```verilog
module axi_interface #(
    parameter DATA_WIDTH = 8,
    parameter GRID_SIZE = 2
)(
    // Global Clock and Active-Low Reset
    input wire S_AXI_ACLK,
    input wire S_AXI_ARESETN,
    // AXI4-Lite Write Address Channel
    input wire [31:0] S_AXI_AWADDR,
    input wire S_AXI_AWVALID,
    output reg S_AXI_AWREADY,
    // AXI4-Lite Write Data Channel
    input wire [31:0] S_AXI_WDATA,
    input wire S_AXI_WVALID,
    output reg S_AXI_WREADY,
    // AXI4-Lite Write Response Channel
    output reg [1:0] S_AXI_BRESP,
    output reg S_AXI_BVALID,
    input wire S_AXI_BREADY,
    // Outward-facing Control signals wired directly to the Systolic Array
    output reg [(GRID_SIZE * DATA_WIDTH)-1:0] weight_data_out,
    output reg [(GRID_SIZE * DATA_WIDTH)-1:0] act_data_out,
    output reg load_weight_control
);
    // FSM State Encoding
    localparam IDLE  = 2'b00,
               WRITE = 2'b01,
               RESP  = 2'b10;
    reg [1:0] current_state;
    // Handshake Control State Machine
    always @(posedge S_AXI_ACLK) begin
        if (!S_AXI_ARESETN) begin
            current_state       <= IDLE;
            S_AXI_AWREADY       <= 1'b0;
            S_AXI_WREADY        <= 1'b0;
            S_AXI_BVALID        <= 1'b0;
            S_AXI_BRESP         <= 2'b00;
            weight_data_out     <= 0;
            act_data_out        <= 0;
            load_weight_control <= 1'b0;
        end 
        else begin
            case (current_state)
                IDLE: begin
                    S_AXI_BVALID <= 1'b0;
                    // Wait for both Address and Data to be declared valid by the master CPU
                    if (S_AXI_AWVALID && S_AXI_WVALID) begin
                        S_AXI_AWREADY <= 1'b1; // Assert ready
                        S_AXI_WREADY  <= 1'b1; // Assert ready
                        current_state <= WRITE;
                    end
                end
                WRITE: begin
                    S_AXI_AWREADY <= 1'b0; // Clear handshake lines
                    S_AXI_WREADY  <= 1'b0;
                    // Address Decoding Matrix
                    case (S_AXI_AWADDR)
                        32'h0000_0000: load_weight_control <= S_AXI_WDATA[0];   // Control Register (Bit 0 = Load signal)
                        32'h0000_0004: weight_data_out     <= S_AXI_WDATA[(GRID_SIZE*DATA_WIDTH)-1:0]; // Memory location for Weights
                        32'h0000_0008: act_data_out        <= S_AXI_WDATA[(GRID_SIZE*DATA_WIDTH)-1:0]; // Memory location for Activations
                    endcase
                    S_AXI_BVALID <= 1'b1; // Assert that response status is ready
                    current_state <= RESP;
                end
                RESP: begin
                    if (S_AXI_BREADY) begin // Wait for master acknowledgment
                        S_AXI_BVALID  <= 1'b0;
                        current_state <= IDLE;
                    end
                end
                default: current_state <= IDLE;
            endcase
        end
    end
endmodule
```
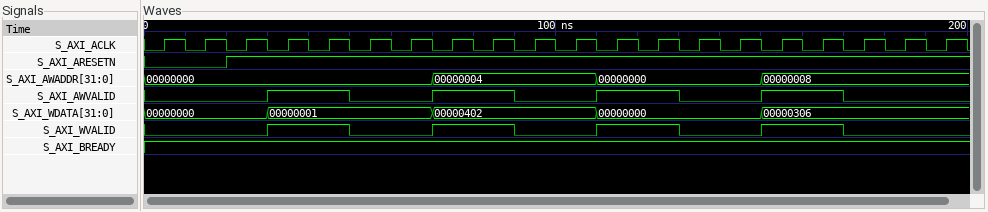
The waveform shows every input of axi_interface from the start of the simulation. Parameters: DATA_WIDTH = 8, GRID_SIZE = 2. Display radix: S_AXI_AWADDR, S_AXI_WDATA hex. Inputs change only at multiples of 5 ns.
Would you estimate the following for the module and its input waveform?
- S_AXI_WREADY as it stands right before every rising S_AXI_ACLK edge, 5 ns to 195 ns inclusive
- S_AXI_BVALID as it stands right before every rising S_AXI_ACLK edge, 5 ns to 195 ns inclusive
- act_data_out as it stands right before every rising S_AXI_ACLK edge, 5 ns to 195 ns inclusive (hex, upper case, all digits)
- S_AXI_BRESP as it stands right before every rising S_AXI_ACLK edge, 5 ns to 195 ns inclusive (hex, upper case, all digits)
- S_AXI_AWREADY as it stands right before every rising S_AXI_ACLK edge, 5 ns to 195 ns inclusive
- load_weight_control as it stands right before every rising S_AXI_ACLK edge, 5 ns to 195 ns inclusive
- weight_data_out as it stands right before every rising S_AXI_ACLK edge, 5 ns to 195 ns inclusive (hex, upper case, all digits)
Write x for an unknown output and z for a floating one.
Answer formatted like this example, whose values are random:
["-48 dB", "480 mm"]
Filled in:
["x 0 0 0 1 0 0 0 1 0 0 0 1 0 0 0 1 0 0 0", "x 0 0 0 0 1 0 0 0 1 0 0 0 1 0 0 0 1 0 0", "x, 0000, 0000, 0000, 0000, 0000, 0000, 0000, 0000, 0000, 0000, 0000, 0000, 0000, 0000, 0000, 0000, 0306, 0306, 0306", "x, 0, 0, 0, 0, 0, 0, 0, 0, 0, 0, 0, 0, 0, 0, 0, 0, 0, 0, 0", "x 0 0 0 1 0 0 0 1 0 0 0 1 0 0 0 1 0 0 0", "x 0 0 0 0 1 1 1 1 1 1 1 1 0 0 0 0 0 0 0", "x, 0000, 0000, 0000, 0000, 0000, 0000, 0000, 0000, 0402, 0402, 0402, 0402, 0402, 0402, 0402, 0402, 0402, 0402, 0402"]
